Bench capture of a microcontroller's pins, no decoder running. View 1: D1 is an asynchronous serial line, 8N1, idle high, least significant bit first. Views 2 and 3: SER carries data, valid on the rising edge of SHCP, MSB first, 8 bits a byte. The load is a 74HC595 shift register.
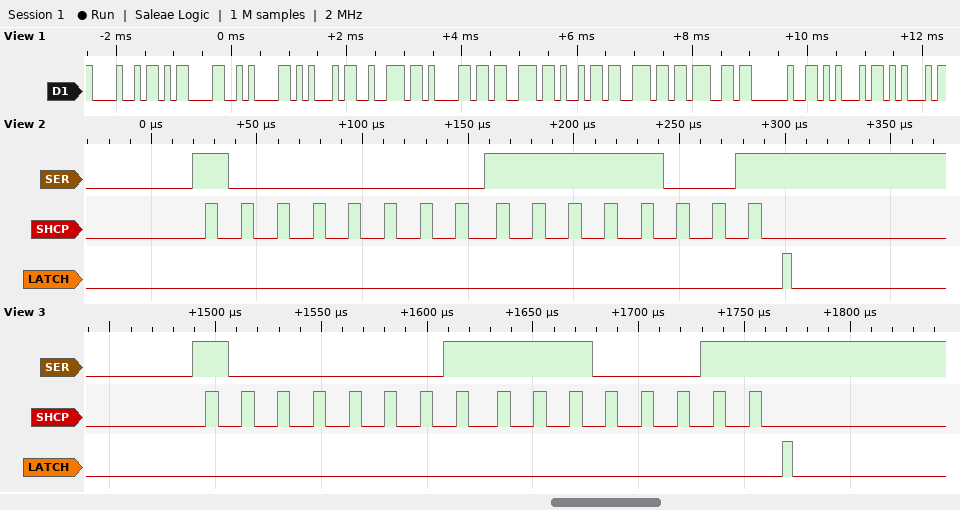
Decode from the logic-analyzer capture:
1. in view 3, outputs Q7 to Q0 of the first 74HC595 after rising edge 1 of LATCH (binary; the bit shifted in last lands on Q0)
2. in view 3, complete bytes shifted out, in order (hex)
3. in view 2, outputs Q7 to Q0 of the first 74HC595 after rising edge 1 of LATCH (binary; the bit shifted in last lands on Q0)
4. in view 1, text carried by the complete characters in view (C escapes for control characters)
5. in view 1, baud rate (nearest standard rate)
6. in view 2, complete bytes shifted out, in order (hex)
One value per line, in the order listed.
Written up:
11100011
81 E3
11111001
"H\r\nErasing EE"
9600 baud
80 F9
